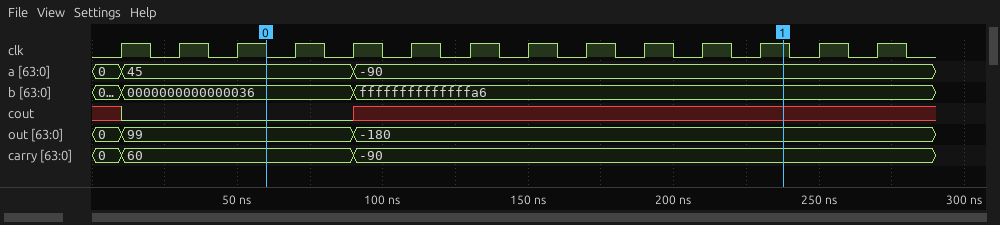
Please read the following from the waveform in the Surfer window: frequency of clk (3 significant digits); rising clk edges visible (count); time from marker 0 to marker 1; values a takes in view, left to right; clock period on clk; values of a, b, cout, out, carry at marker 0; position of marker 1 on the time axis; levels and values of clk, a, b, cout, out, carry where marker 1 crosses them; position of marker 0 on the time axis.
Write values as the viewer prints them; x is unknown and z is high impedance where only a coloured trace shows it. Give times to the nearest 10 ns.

50.0 MHz
14
180 ns
0, 45, -90
20 ns
a=45, b=0000000000000036, cout=0, out=99, carry=60
240 ns
clk=1, a=-90, b=ffffffffffffffa6, cout=x, out=-180, carry=-90
60 ns
